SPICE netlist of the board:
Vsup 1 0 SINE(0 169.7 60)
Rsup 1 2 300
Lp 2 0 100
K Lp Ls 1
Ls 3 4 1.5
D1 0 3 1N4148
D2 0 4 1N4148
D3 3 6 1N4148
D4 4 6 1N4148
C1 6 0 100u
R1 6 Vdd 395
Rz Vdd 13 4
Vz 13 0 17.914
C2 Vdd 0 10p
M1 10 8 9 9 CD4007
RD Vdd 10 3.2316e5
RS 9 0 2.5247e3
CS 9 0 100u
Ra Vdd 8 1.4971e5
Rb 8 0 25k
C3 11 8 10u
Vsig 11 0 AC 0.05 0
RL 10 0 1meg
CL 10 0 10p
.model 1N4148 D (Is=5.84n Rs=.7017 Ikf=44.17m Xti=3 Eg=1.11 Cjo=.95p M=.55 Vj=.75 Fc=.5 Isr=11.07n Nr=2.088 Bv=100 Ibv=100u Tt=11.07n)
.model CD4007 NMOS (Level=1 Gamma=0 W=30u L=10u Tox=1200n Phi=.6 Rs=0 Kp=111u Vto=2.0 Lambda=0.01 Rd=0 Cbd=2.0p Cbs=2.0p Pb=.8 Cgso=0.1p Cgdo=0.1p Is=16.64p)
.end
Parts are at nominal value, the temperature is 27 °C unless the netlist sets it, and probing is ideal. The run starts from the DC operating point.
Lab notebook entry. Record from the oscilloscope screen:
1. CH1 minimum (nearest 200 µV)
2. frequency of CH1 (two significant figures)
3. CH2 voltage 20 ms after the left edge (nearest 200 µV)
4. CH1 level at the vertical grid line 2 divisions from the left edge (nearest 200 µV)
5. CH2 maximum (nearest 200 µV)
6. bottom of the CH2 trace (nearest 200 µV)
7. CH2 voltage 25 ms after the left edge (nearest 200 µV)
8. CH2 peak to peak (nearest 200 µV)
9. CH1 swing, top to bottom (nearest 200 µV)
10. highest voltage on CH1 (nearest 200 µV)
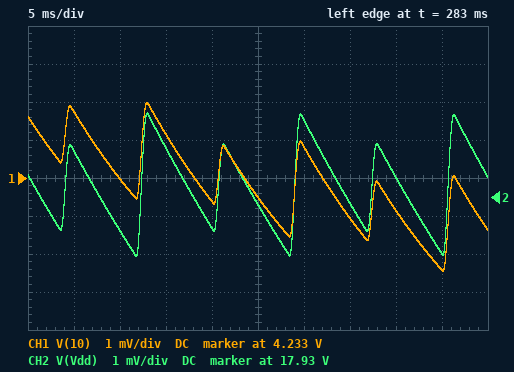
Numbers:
4.2306 V
120 Hz
17.9292 V
4.2330 V
17.9322 V
17.9284 V
17.9298 V
3.8 mV
4.4 mV
4.2350 V
